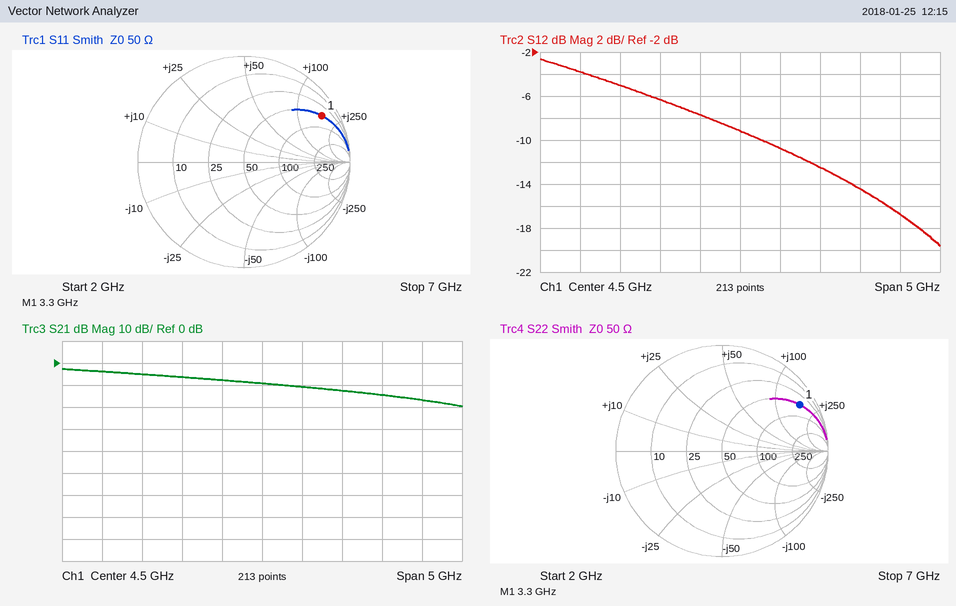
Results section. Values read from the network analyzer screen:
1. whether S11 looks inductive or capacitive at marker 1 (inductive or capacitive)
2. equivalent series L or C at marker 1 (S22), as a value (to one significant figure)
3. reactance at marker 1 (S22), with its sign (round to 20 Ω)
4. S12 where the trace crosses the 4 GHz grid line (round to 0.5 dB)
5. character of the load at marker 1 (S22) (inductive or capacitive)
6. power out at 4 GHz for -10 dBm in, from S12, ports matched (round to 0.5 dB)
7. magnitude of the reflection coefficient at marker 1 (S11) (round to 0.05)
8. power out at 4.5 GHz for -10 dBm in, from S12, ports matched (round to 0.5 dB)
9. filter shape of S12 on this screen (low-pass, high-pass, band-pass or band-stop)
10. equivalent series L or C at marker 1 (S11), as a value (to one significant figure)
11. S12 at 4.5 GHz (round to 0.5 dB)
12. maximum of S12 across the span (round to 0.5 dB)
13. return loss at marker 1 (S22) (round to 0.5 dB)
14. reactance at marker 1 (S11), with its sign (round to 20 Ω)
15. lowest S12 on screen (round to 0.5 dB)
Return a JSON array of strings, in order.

["inductive", "8 nH", "+160 Ω", "-7.5 dB", "inductive", "-17.5 dBm", "0.85", "-19.0 dBm", "low-pass", "8 nH", "-9.0 dB", "-2.5 dB", "1.5 dB", "+160 Ω", "-19.5 dB"]
